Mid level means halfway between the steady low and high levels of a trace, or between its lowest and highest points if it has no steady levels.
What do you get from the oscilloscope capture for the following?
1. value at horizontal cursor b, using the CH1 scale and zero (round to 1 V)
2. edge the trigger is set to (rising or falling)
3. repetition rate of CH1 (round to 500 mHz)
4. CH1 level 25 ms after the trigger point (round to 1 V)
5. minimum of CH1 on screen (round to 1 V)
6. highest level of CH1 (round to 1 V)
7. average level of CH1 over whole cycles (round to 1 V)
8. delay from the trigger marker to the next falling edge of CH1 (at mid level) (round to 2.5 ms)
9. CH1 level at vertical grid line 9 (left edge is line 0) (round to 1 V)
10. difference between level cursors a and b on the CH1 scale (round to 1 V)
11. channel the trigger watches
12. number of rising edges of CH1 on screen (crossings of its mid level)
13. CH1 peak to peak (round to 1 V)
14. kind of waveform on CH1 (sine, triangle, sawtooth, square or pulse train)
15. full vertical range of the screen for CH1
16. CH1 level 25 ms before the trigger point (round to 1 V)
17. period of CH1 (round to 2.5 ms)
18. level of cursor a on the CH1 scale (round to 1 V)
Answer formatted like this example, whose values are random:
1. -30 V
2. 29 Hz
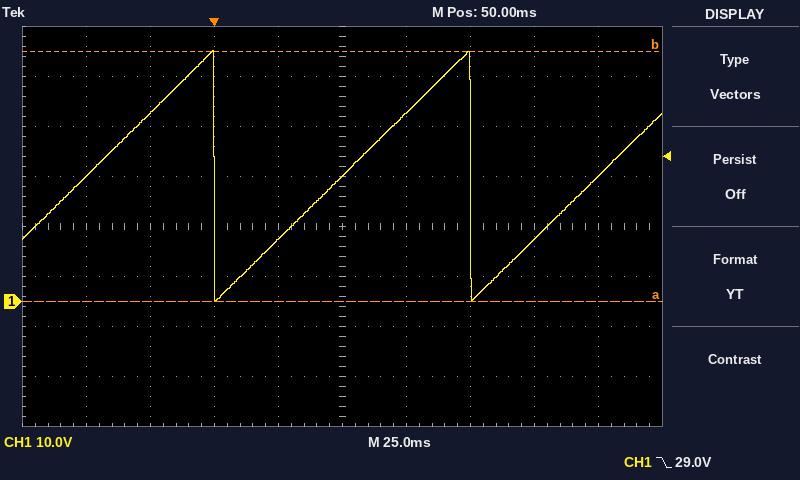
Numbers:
1. 50 V
2. falling
3. 10.0 Hz
4. 12 V
5. 0 V
6. 50 V
7. 25 V
8. 100.0 ms
9. 25 V
10. 50 V
11. CH1
12. 3
13. 50 V
14. sawtooth
15. 80 V
16. 38 V
17. 100.0 ms
18. 0 V
